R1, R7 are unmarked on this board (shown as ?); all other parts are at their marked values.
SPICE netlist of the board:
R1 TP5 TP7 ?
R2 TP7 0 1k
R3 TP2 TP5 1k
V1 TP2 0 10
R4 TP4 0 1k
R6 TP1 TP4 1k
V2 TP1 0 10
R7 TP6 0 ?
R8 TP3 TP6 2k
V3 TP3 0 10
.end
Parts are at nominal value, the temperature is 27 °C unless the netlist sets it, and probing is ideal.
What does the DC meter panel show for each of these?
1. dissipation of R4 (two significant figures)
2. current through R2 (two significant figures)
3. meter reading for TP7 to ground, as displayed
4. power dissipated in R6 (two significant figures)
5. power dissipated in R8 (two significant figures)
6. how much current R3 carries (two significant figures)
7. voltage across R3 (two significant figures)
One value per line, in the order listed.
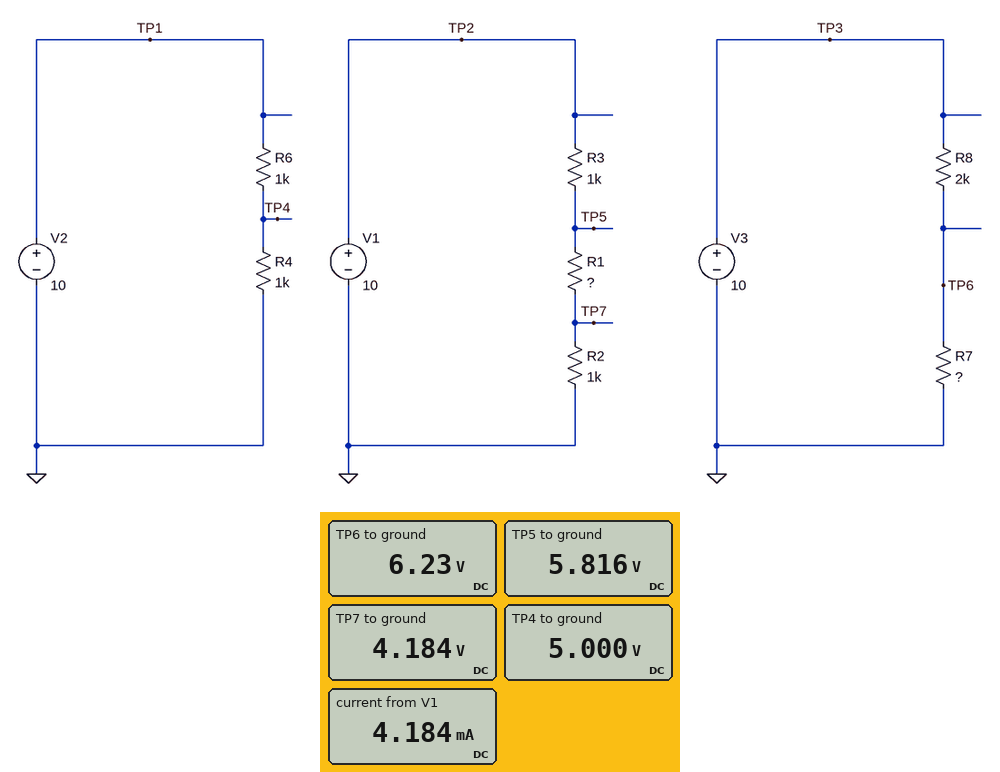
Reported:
25 mW
4.2 mA
4.184 V
25 mW
7.1 mW
4.2 mA
4.2 V
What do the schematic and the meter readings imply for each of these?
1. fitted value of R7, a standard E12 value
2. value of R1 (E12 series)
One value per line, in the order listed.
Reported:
3.3 kΩ
390 Ω
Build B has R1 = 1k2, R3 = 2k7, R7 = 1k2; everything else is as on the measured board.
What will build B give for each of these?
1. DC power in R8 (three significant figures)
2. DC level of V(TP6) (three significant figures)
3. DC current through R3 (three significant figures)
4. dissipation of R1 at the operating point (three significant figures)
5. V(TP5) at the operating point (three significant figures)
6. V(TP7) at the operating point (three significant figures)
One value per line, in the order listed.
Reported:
19.5 mW
3.75 V
2.04 mA
5.00 mW
4.49 V
2.04 V
